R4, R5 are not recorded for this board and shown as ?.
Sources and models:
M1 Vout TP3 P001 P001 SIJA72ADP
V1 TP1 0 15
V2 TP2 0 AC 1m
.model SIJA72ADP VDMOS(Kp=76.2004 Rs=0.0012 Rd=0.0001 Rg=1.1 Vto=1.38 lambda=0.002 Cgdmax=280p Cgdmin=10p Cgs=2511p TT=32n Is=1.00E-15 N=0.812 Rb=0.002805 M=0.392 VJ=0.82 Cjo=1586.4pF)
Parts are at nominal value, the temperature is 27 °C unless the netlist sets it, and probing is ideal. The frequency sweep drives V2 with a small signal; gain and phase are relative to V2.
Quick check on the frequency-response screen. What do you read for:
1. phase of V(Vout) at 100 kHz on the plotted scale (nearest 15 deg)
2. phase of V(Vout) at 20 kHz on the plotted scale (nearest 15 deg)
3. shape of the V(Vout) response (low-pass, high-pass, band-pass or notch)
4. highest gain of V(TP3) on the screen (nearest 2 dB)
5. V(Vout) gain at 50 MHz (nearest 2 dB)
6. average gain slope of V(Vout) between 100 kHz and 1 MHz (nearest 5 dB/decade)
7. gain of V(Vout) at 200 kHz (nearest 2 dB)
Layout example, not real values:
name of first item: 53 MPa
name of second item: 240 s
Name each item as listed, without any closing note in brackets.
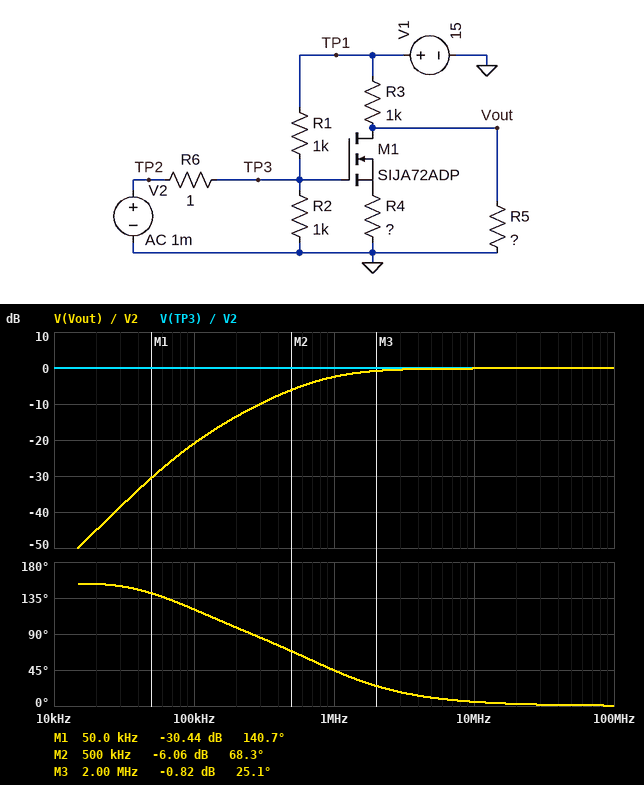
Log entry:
phase of V(Vout) at 100 kHz on the plotted scale: 120 deg
phase of V(Vout) at 20 kHz on the plotted scale: 150 deg
shape of the V(Vout) response: high-pass
highest gain of V(TP3) on the screen: 0 dB
V(Vout) gain at 50 MHz: 0 dB
average gain slope of V(Vout) between 100 kHz and 1 MHz: 20 dB/decade
gain of V(Vout) at 200 kHz: -14 dB
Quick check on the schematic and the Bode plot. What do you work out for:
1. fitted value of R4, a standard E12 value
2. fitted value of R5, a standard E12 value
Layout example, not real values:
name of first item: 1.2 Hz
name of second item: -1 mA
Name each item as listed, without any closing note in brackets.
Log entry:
fitted value of R4, a standard E12 value: 560 Ω
fitted value of R5, a standard E12 value: 470 Ω
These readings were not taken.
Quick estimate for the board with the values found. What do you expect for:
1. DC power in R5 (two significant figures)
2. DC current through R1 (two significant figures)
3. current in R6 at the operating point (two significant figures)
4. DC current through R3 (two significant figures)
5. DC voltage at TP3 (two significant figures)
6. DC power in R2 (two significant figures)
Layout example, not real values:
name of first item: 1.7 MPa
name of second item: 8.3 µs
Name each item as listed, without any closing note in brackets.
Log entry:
DC power in R5: 49 mW
DC current through R1: 15 mA
current in R6 at the operating point: 15 mA
DC current through R3: 10 mA
DC voltage at TP3: 15 mV
DC power in R2: 220 nW
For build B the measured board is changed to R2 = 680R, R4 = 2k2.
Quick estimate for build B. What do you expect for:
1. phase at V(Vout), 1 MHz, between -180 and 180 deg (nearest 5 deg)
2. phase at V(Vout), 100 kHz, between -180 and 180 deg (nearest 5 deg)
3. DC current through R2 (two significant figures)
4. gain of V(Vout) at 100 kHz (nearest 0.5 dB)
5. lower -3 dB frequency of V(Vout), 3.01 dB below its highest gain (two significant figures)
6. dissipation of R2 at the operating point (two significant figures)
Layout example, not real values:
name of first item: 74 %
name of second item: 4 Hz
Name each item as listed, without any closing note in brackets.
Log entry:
phase at V(Vout), 1 MHz, between -180 and 180 deg: 40 deg
phase at V(Vout), 100 kHz, between -180 and 180 deg: 95 deg
DC current through R2: 22 µA
gain of V(Vout) at 100 kHz: -18.5 dB
lower -3 dB frequency of V(Vout), 3.01 dB below its highest gain: 820 kHz
dissipation of R2 at the operating point: 330 nW
